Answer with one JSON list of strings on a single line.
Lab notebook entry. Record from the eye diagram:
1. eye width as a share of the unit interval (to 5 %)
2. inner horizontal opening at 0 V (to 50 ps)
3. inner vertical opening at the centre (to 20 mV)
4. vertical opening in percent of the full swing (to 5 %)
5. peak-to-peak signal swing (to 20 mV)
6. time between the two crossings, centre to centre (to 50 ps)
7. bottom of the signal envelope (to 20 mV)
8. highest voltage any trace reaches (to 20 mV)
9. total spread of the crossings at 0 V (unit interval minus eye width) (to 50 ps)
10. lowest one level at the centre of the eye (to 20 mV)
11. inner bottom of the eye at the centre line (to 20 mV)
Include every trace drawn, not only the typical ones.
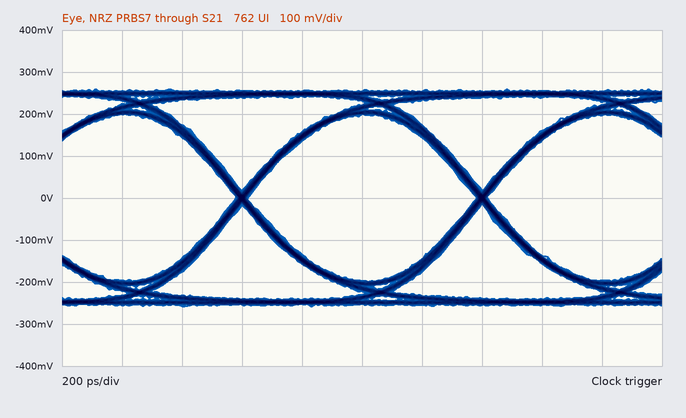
["95 %", "750 ps", "400 mV", "75 %", "520 mV", "800 ps", "-260 mV", "260 mV", "50 ps", "200 mV", "-200 mV"]
